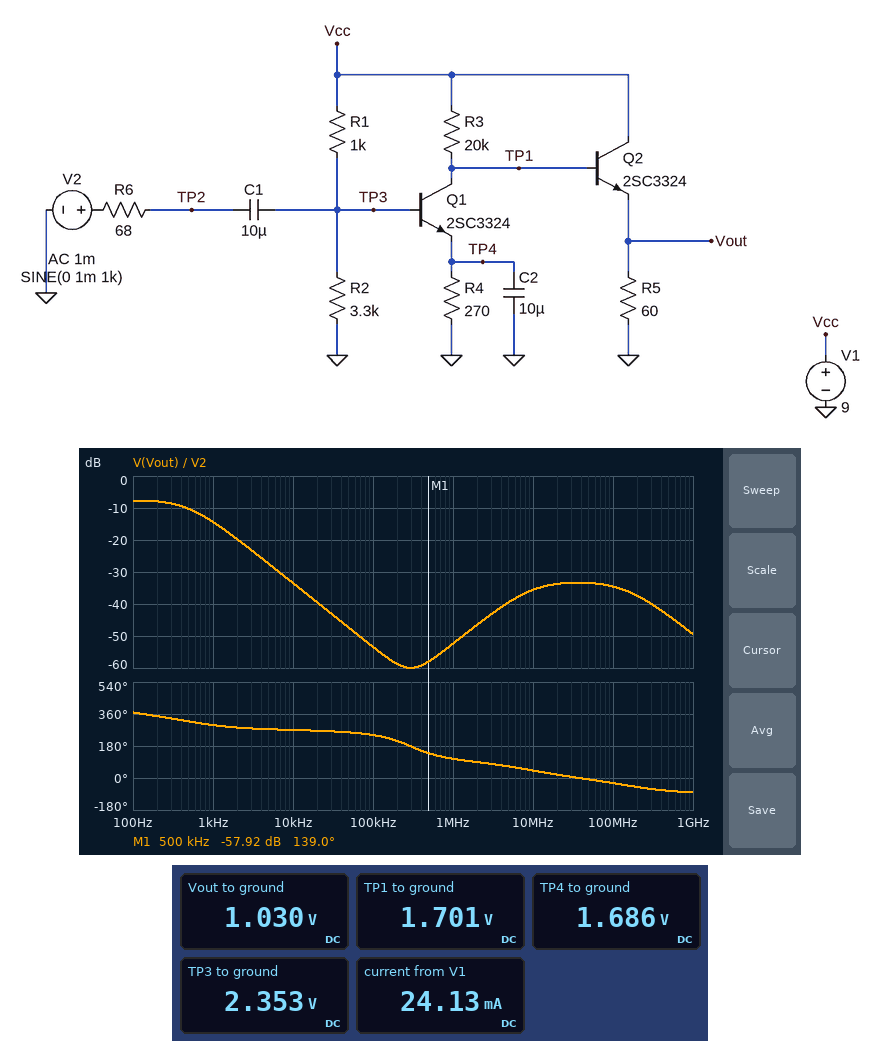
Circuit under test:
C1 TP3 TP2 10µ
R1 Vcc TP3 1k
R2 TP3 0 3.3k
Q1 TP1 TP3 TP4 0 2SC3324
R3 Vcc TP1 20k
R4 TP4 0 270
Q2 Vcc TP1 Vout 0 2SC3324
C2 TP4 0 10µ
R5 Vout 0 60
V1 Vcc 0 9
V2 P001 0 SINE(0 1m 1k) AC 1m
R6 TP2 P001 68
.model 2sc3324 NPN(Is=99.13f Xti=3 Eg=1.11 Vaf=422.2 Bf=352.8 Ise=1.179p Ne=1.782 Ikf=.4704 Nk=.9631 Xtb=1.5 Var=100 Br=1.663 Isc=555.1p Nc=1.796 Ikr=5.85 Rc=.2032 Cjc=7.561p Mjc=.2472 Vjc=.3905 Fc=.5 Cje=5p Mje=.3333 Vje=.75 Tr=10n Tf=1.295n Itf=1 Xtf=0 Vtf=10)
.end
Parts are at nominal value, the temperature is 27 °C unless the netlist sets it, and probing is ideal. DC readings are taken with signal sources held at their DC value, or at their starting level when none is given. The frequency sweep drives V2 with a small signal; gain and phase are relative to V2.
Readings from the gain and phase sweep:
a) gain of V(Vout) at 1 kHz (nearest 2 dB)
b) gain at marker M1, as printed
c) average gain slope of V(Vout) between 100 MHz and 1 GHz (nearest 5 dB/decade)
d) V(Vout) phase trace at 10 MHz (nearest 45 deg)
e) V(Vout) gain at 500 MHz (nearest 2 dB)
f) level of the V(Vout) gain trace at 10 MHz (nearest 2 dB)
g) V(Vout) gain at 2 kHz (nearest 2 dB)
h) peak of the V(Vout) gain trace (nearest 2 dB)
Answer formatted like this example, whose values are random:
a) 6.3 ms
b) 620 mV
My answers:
a) -14 dB
b) -57.92 dB
c) -15 dB/decade
d) 45 deg
e) -44 dB
f) -36 dB
g) -20 dB
h) -8 dB
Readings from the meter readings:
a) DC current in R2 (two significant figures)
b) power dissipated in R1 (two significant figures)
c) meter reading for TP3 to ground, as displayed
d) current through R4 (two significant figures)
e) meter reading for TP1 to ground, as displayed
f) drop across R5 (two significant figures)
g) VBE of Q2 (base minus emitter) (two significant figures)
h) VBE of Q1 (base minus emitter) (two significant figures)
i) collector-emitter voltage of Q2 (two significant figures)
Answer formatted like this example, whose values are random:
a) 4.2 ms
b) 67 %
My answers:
a) 710 µA
b) 44 mW
c) 2.353 V
d) 6.2 mA
e) 1.701 V
f) 1.0 V
g) 670 mV
h) 670 mV
i) 8.0 V
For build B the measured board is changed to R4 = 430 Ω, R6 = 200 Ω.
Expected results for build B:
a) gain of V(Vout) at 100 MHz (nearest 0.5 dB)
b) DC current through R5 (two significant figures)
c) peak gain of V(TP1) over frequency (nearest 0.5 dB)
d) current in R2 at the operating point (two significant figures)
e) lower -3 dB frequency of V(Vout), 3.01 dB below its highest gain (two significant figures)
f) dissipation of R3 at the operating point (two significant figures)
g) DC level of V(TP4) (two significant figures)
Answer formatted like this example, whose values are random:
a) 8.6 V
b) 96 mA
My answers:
a) -42.5 dB
b) 27 mA
c) -9.0 dB
d) 900 µA
e) 20 Hz
f) 2.2 mW
g) 2.3 V
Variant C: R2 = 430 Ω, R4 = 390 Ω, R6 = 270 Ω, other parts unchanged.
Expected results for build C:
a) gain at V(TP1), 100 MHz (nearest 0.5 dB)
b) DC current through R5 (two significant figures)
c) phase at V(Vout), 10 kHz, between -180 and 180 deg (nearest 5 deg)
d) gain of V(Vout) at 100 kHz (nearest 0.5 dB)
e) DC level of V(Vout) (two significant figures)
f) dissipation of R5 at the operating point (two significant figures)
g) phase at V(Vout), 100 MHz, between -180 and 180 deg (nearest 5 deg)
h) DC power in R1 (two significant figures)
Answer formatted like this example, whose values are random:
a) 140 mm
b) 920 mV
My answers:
a) -40.5 dB
b) 9.7 mA
c) -110 deg
d) -53.0 dB
e) 580 mV
f) 5.7 mW
g) -30 deg
h) 51 mW
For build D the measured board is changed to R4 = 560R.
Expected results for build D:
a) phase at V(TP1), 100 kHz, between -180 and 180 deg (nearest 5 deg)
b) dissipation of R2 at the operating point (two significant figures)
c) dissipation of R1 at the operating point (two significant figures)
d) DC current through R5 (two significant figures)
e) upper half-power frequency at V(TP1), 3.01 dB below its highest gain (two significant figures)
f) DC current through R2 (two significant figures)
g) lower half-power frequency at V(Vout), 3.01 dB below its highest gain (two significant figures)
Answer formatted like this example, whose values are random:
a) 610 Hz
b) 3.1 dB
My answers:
a) -135 deg
b) 3.4 mW
c) 32 mW
d) 34 mA
e) 500 Hz
f) 1.0 mA
g) 22 Hz
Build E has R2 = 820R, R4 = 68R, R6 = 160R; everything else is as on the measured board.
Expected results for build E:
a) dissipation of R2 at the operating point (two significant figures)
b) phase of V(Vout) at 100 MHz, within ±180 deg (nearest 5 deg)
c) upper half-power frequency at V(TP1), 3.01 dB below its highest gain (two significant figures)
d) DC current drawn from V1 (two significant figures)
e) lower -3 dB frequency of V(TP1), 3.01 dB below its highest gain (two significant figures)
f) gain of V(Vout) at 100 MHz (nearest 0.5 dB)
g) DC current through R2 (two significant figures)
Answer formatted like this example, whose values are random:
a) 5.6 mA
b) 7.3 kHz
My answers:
a) 1.6 mW
b) 40 deg
c) 510 Hz
d) 8.3 mA
e) 51 Hz
f) -54.0 dB
g) 1.4 mA
